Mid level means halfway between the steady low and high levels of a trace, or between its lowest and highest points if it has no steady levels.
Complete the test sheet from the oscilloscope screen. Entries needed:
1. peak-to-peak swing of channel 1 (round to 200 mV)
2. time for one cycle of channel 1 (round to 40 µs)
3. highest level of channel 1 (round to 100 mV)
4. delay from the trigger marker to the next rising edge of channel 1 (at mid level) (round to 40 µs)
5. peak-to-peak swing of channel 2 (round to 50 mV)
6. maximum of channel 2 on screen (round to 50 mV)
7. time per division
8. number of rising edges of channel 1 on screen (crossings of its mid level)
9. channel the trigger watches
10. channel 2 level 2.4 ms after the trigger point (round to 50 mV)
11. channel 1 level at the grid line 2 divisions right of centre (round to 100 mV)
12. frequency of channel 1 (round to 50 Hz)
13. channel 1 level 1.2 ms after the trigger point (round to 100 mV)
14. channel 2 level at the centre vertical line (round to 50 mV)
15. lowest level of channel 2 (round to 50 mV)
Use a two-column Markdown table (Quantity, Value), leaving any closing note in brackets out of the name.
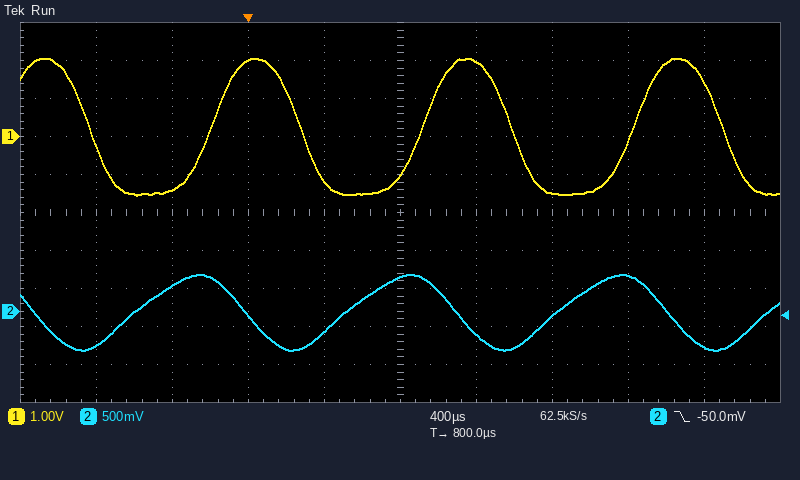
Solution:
| Quantity | Value |
|---|---|
| peak-to-peak swing of channel 1 | 3.6 V |
| time for one cycle of channel 1 | 1.12 ms |
| highest level of channel 1 | 2.1 V |
| delay from the trigger marker to the next rising edge of channel 1 (at mid level) | 920 µs |
| peak-to-peak swing of channel 2 | 1.00 V |
| maximum of channel 2 on screen | 500 mV |
| time per division | 400 µs |
| number of rising edges of channel 1 on screen | 3 |
| channel the trigger watches | channel 2 |
| channel 2 level 2.4 ms after the trigger point | -450 mV |
| channel 1 level at the grid line 2 divisions right of centre | -1.5 V |
| frequency of channel 1 | 900 Hz |
| channel 1 level 1.2 ms after the trigger point | 2.0 V |
| channel 2 level at the centre vertical line | 450 mV |
| lowest level of channel 2 | -500 mV |
